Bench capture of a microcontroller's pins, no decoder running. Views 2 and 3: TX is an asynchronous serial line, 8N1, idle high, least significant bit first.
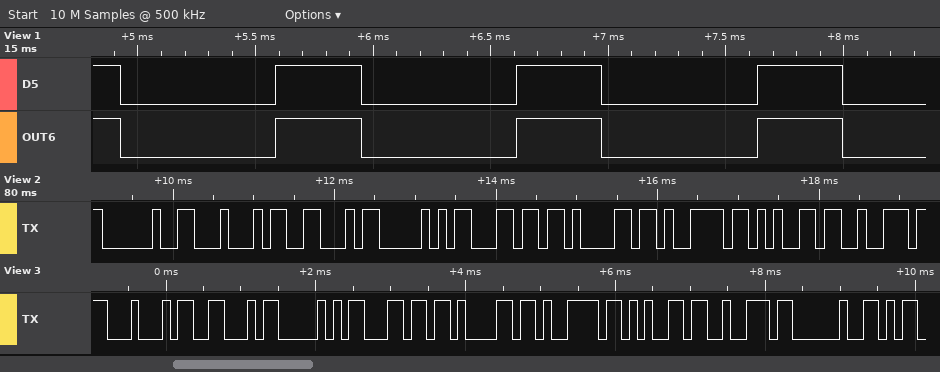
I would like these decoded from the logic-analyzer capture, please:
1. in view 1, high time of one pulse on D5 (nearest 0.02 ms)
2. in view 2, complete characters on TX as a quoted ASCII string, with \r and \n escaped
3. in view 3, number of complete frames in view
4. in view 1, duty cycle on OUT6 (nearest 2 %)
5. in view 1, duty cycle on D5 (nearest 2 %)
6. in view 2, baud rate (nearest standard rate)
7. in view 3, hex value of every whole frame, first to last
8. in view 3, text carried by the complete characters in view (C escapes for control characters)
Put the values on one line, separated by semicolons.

0.36 ms; " DFPlayer"; 9; 36 %; 36 %; 9600 baud; 44 46 50 6C 61 79 65 72 20; "DFPlayer "
